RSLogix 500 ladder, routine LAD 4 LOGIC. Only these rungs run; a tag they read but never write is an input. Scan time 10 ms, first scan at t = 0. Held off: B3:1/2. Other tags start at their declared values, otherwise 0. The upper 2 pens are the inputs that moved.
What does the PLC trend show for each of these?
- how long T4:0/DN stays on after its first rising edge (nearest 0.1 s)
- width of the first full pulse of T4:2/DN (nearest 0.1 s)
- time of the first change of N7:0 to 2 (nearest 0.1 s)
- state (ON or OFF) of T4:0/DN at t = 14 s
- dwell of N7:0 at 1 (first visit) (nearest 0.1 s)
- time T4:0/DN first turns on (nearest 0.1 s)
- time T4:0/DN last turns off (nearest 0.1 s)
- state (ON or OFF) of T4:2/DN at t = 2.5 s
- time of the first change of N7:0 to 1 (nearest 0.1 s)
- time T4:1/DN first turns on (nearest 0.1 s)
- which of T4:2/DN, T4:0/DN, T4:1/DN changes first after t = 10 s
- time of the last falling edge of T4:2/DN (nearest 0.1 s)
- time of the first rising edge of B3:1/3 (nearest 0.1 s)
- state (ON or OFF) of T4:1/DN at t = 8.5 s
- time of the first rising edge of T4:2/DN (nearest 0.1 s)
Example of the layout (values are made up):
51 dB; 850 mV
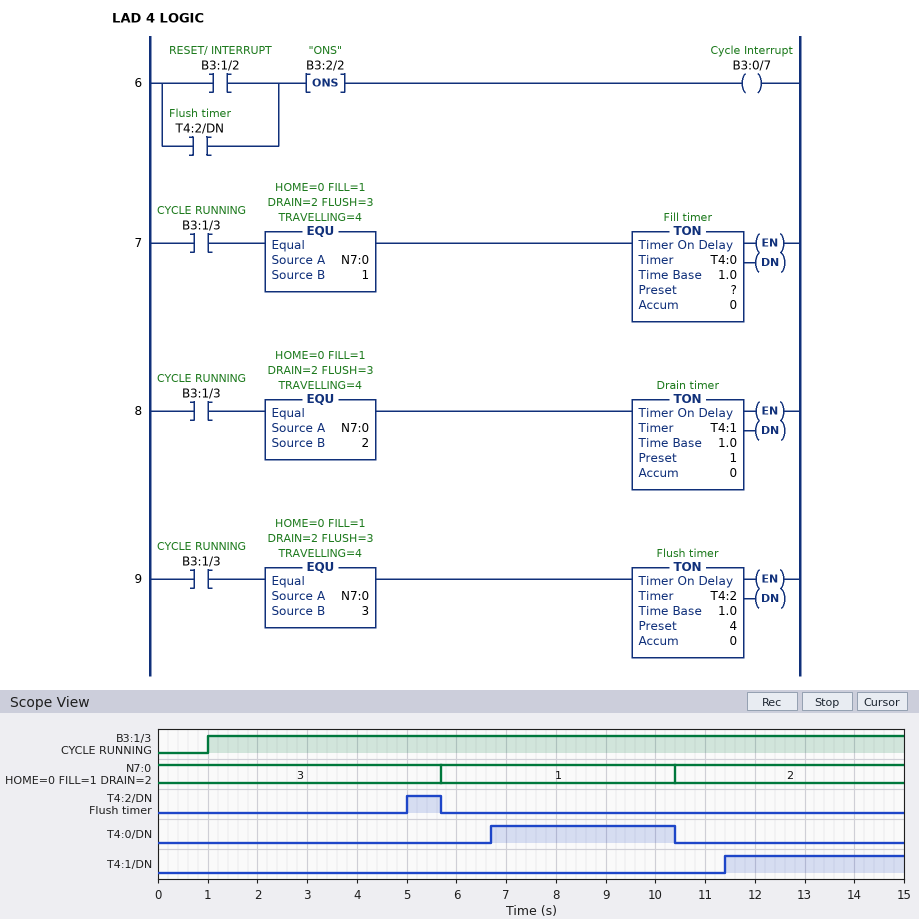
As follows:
3.7 s; 0.7 s; 10.4 s; OFF; 4.7 s; 6.7 s; 10.4 s; OFF; 5.7 s; 11.4 s; T4:0/DN; 5.7 s; 1.0 s; OFF; 5.0 s
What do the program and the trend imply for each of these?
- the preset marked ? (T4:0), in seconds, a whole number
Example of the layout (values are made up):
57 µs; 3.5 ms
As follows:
1 s
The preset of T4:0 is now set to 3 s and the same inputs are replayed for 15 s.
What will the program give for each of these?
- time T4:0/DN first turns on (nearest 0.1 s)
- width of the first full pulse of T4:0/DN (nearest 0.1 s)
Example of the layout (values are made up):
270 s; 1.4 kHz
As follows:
8.7 s; 1.7 s
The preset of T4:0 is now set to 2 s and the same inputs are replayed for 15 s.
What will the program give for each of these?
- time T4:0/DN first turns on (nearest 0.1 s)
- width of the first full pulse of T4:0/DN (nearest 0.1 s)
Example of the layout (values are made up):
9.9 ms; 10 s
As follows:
7.7 s; 2.7 s
